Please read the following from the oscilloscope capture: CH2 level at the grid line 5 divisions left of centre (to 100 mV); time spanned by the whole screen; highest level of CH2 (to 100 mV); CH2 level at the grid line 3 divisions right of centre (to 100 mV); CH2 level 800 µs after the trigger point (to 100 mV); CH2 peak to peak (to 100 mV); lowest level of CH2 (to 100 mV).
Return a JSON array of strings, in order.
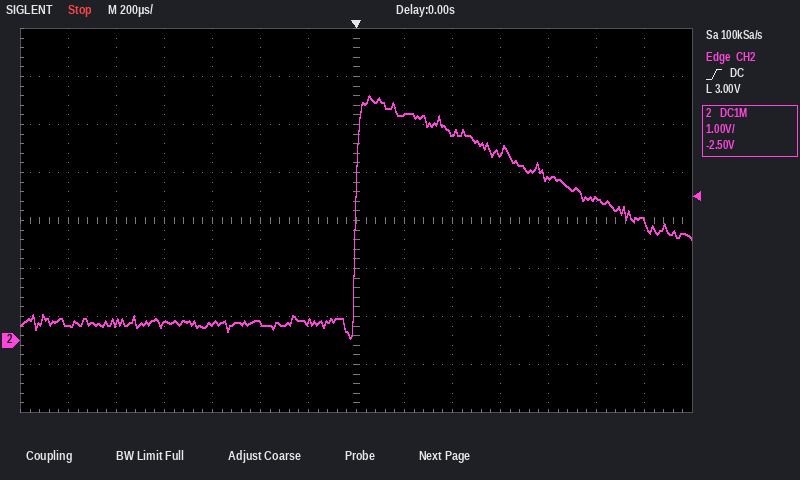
["400 mV", "2.8 ms", "5.1 V", "3.9 V", "3.4 V", "5.1 V", "0.0 V"]
